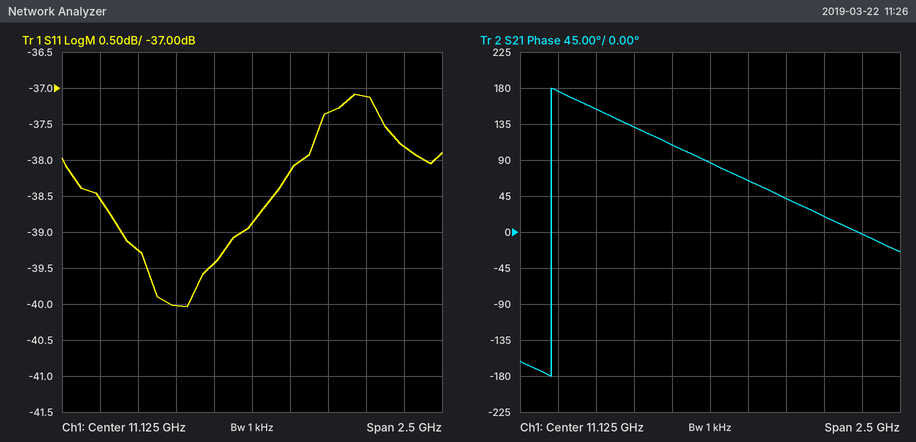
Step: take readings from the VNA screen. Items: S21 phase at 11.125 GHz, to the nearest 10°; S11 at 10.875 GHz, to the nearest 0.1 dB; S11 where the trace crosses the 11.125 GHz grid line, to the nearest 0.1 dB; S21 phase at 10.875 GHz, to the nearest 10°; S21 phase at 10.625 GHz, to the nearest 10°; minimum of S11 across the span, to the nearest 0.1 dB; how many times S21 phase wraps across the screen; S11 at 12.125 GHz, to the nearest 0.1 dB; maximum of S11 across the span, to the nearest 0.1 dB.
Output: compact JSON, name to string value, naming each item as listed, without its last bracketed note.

{"S21 phase at 11.125 GHz, to the nearest 10°": "90°", "S11 at 10.875 GHz, to the nearest 0.1 dB": "-39.4 dB", "S11 where the trace crosses the 11.125 GHz grid line, to the nearest 0.1 dB": "-38.9 dB", "S21 phase at 10.875 GHz, to the nearest 10°": "110°", "S21 phase at 10.625 GHz, to the nearest 10°": "130°", "minimum of S11 across the span, to the nearest 0.1 dB": "-40.0 dB", "how many times S21 phase wraps across the screen": "1", "S11 at 12.125 GHz, to the nearest 0.1 dB": "-37.8 dB", "maximum of S11 across the span, to the nearest 0.1 dB": "-37.1 dB"}
